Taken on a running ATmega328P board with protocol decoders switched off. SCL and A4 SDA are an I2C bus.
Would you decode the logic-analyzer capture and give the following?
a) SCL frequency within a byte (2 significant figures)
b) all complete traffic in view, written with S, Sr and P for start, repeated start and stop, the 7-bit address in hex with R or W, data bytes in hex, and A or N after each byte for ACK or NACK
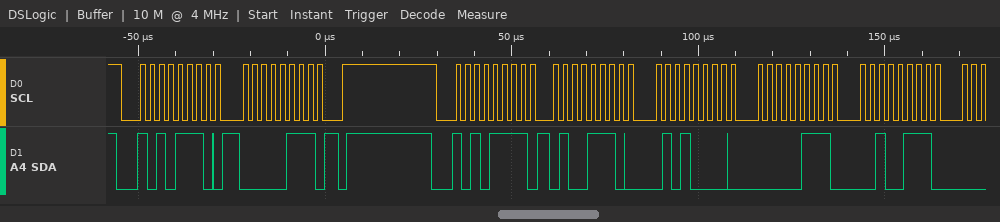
400 kHz
S 57W A 07 A P S 57R A 4E A 50 A 07 A 27 A
